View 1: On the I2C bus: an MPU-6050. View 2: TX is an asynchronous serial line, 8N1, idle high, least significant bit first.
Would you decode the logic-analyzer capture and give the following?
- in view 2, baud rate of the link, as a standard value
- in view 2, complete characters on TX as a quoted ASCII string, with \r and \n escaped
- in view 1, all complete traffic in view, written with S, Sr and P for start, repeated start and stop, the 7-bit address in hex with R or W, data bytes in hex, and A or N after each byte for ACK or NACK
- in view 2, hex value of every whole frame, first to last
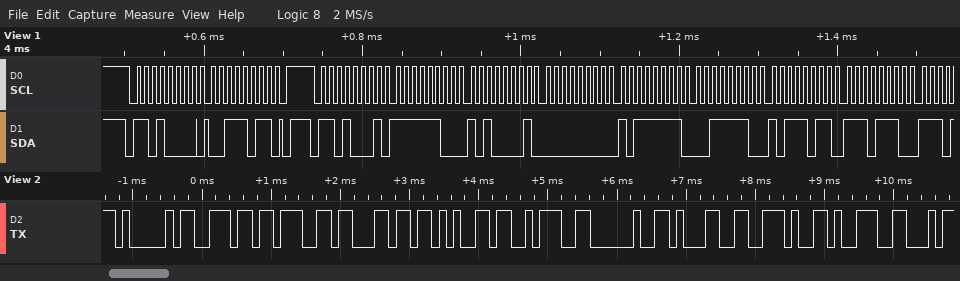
9600 baud
"Angle: 1.9"
S 68W A 3B A P S 68R A FC A A1 A 00 A BF A 3E A BB A EE A
41 6E 67 6C 65 3A 20 31 2E 39
